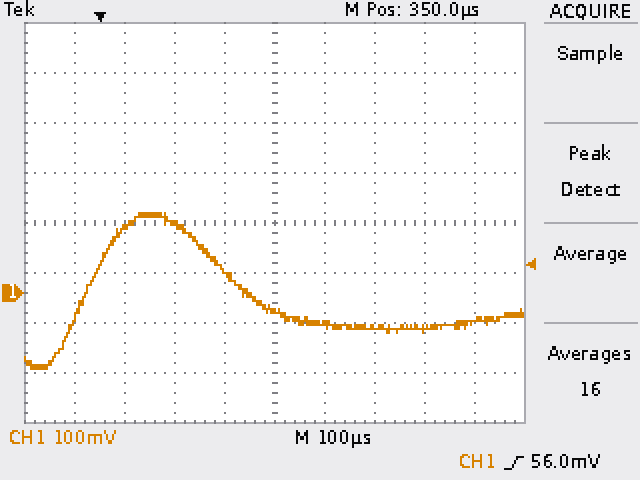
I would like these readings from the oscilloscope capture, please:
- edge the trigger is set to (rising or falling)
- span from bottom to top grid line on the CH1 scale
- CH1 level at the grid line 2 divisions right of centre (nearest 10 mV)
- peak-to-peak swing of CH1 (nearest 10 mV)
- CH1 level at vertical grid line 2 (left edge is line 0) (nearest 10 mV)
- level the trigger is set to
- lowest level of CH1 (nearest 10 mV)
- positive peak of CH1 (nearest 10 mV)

rising
800 mV
-70 mV
310 mV
130 mV
56.0 mV
-150 mV
160 mV
